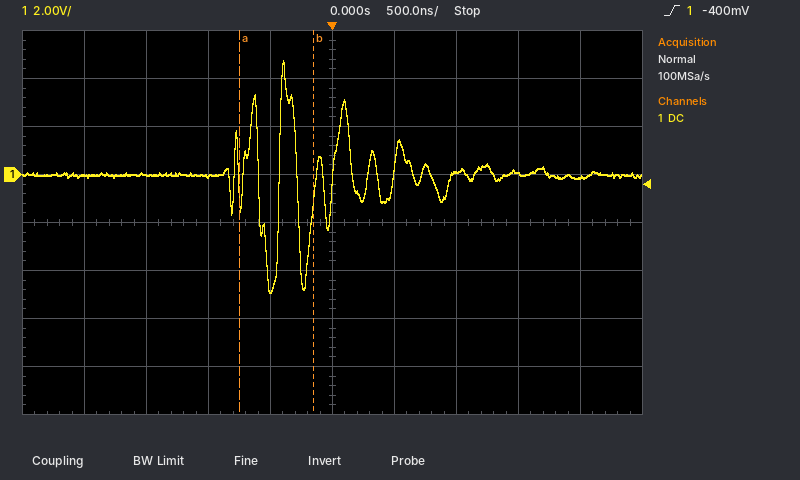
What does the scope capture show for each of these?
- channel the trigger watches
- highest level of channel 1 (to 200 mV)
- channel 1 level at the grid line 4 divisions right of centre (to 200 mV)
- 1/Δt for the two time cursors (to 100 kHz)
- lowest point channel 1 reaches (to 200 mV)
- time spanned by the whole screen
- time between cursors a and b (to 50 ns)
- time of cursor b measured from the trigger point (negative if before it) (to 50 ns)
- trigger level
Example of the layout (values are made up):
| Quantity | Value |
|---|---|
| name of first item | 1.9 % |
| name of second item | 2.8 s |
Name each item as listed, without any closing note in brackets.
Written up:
| Quantity | Value |
|---|---|
| channel the trigger watches | channel 1 |
| highest level of channel 1 | 4.8 V |
| channel 1 level at the grid line 4 divisions right of centre | -200 mV |
| 1/Δt for the two time cursors | 1.7 MHz |
| lowest point channel 1 reaches | -5.0 V |
| time spanned by the whole screen | 5 µs |
| time between cursors a and b | 600 ns |
| time of cursor b measured from the trigger point (negative if before it) | -150 ns |
| trigger level | -400 mV |
